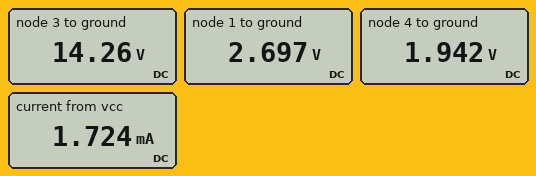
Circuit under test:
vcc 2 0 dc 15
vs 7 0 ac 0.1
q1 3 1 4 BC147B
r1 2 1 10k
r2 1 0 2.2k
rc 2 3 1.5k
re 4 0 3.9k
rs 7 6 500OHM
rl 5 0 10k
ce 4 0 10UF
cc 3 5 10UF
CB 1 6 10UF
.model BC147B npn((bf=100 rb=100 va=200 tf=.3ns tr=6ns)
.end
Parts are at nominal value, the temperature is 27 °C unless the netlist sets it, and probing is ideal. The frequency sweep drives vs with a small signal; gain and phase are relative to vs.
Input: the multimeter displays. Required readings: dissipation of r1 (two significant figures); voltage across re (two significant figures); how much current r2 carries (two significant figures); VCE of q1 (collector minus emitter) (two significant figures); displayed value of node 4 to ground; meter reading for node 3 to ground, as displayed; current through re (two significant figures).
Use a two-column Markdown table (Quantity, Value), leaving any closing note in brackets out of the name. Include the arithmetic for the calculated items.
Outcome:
| Quantity | Value |
|---|---|
| dissipation of r1 | (15 V - 2.697 V)^2 / 10 kΩ = 15 mW |
| voltage across re | 1.942 V = 1.9 V |
| how much current r2 carries | (2.697 V) / 2.2 kΩ = 1.2 mA |
| VCE of q1 (collector minus emitter) | 14.26 V - 1.942 V = 12 V |
| displayed value of node 4 to ground | 1.942 V |
| meter reading for node 3 to ground, as displayed | 14.26 V |
| current through re | (1.942 V) / 3.9 kΩ = 500 µA |
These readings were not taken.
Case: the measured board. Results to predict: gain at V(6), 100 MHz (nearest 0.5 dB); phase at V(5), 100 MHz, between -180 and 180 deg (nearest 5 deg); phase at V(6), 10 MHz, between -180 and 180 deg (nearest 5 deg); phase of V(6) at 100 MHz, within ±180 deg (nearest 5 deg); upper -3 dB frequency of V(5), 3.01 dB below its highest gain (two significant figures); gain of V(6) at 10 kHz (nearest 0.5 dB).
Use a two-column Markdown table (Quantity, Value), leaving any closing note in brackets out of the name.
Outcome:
| Quantity | Value |
|---|---|
| gain at V(6), 100 MHz | -8.0 dB |
| phase at V(5), 100 MHz, between -180 and 180 deg | 120 deg |
| phase at V(6), 10 MHz, between -180 and 180 deg | -5 deg |
| phase of V(6) at 100 MHz, within ±180 deg | -40 deg |
| upper -3 dB frequency of V(5), 3.01 dB below its highest gain | 62 MHz |
| gain of V(6) at 10 kHz | -2.5 dB |
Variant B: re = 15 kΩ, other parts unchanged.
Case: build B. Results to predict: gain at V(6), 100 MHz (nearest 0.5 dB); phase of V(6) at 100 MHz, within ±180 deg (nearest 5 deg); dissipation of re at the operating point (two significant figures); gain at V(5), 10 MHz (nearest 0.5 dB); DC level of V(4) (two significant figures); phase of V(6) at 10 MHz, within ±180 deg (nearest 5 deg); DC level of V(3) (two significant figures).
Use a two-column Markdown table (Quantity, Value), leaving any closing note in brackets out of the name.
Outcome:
| Quantity | Value |
|---|---|
| gain at V(6), 100 MHz | -3.0 dB |
| phase of V(6) at 100 MHz, within ±180 deg | -20 deg |
| dissipation of re at the operating point | 260 µW |
| gain at V(5), 10 MHz | 14.0 dB |
| DC level of V(4) | 2.0 V |
| phase of V(6) at 10 MHz, within ±180 deg | 0 deg |
| DC level of V(3) | 15 V |
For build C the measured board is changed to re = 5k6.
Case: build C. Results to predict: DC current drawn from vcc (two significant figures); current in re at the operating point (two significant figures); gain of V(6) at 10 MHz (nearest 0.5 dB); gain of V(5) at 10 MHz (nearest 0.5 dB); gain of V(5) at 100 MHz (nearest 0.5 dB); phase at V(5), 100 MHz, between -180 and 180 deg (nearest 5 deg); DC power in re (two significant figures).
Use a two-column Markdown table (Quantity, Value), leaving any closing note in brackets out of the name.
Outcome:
| Quantity | Value |
|---|---|
| DC current drawn from vcc | 1.6 mA |
| current in re at the operating point | 350 µA |
| gain of V(6) at 10 MHz | -2.5 dB |
| gain of V(5) at 10 MHz | 22.0 dB |
| gain of V(5) at 100 MHz | 18.5 dB |
| phase at V(5), 100 MHz, between -180 and 180 deg | 130 deg |
| DC power in re | 680 µW |
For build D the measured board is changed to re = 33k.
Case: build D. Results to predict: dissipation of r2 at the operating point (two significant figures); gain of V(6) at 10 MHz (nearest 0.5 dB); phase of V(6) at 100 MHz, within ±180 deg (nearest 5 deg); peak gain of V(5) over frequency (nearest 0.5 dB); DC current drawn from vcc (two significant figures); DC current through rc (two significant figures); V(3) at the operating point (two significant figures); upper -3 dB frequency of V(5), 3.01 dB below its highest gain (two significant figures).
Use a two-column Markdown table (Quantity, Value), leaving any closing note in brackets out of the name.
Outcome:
| Quantity | Value |
|---|---|
| dissipation of r2 at the operating point | 3.3 mW |
| gain of V(6) at 10 MHz | -2.0 dB |
| phase of V(6) at 100 MHz, within ±180 deg | -10 deg |
| peak gain of V(5) over frequency | 7.5 dB |
| DC current drawn from vcc | 1.3 mA |
| DC current through rc | 60 µA |
| V(3) at the operating point | 15 V |
| upper -3 dB frequency of V(5), 3.01 dB below its highest gain | 470 MHz |
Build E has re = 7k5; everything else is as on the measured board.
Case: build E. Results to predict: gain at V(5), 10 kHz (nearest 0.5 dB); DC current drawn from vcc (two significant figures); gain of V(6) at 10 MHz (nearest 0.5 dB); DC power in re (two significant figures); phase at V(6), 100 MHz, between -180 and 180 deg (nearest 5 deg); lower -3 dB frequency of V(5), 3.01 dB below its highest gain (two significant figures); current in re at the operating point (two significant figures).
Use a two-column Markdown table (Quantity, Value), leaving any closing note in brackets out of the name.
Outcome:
| Quantity | Value |
|---|---|
| gain at V(5), 10 kHz | 20.0 dB |
| DC current drawn from vcc | 1.5 mA |
| gain of V(6) at 10 MHz | -2.5 dB |
| DC power in re | 510 µW |
| phase at V(6), 100 MHz, between -180 and 180 deg | -30 deg |
| lower -3 dB frequency of V(5), 3.01 dB below its highest gain | 160 Hz |
| current in re at the operating point | 260 µA |
